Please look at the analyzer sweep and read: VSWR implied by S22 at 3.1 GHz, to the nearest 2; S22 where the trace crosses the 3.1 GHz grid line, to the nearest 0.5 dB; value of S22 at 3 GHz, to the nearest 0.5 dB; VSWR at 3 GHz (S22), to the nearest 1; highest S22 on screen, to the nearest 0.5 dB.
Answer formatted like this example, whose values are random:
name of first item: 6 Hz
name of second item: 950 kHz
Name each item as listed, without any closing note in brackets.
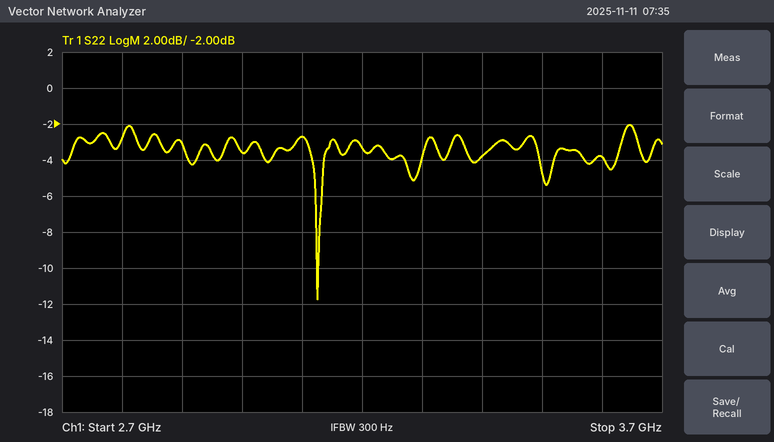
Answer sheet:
VSWR implied by S22 at 3.1 GHz, to the nearest 2: 6
S22 where the trace crosses the 3.1 GHz grid line, to the nearest 0.5 dB: -2.5 dB
value of S22 at 3 GHz, to the nearest 0.5 dB: -3.5 dB
VSWR at 3 GHz (S22), to the nearest 1: 5
highest S22 on screen, to the nearest 0.5 dB: -2.0 dB
